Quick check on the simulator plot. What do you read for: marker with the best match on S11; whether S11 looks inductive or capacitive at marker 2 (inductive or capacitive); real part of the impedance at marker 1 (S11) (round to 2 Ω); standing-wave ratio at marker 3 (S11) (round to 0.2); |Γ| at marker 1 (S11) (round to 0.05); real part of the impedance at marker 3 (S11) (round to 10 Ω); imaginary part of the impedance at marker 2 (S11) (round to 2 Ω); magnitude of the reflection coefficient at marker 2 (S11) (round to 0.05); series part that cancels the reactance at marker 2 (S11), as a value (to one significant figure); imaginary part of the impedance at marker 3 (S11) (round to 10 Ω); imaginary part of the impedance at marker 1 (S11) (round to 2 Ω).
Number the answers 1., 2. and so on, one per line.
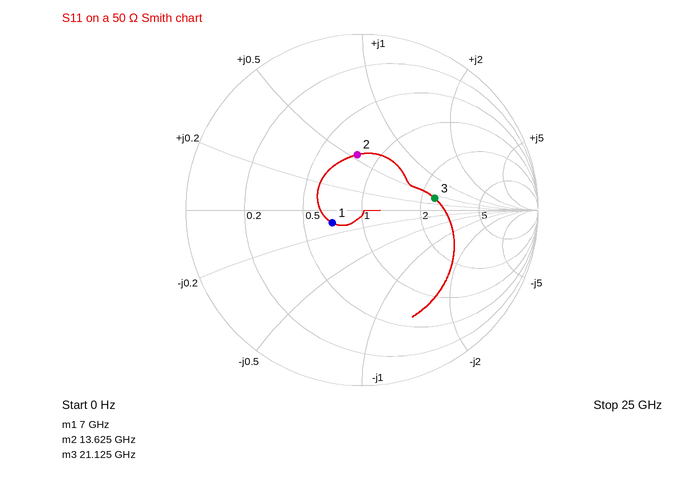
1. marker 1
2. inductive
3. 36 Ω
4. 2.4
5. 0.20
6. 120 Ω
7. +28 Ω
8. 0.30
9. 400 fF
10. +20 Ω
11. -6 Ω
